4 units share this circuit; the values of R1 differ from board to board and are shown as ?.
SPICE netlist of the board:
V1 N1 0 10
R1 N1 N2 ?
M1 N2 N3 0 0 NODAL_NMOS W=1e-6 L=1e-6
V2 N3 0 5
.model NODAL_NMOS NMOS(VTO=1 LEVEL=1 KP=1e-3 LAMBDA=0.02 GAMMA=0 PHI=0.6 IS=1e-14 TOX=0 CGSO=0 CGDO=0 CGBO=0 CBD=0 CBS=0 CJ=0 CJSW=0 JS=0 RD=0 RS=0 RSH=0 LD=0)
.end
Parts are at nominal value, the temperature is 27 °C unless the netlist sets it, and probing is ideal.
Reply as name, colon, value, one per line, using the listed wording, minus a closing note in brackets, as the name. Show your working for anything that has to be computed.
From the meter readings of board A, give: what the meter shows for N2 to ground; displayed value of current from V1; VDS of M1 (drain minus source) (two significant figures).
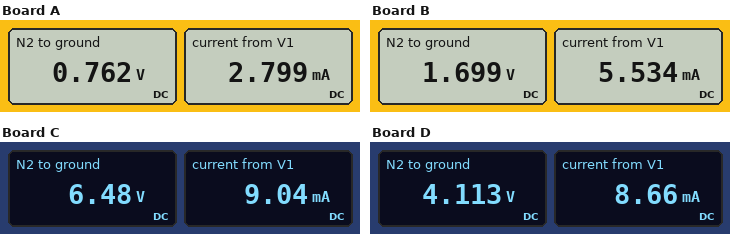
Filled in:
what the meter shows for N2 to ground: 0.762 V
displayed value of current from V1: 2.799 mA
VDS of M1 (drain minus source): 762 mV = 760 mV
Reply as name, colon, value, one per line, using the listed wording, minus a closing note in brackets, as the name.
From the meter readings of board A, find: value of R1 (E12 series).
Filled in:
value of R1: 3.3 kΩ
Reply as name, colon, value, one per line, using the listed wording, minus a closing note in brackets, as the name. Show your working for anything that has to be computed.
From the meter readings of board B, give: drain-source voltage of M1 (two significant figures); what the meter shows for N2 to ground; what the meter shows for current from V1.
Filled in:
drain-source voltage of M1: 1.699 V = 1.7 V
what the meter shows for N2 to ground: 1.699 V
what the meter shows for current from V1: 5.534 mA
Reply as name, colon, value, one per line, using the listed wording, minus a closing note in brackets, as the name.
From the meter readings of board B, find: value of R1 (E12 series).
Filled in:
value of R1: 1.5 kΩ
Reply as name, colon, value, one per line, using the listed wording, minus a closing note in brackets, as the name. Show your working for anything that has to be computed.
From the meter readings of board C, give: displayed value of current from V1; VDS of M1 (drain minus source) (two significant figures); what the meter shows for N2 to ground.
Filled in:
displayed value of current from V1: 9.04 mA
VDS of M1 (drain minus source): 6.48 V = 6.5 V
what the meter shows for N2 to ground: 6.48 V
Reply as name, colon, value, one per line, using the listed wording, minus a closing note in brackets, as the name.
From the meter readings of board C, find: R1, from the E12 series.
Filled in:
R1, from the E12 series: 390 Ω
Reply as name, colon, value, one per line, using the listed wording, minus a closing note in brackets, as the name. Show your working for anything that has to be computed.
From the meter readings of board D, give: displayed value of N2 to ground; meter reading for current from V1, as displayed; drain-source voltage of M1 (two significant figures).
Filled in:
displayed value of N2 to ground: 4.113 V
meter reading for current from V1, as displayed: 8.66 mA
drain-source voltage of M1: 4.113 V = 4.1 V
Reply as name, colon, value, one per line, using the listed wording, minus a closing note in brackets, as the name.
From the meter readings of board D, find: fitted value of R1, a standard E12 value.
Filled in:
fitted value of R1, a standard E12 value: 680 Ω
